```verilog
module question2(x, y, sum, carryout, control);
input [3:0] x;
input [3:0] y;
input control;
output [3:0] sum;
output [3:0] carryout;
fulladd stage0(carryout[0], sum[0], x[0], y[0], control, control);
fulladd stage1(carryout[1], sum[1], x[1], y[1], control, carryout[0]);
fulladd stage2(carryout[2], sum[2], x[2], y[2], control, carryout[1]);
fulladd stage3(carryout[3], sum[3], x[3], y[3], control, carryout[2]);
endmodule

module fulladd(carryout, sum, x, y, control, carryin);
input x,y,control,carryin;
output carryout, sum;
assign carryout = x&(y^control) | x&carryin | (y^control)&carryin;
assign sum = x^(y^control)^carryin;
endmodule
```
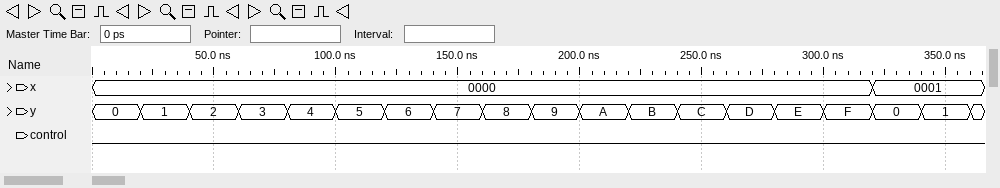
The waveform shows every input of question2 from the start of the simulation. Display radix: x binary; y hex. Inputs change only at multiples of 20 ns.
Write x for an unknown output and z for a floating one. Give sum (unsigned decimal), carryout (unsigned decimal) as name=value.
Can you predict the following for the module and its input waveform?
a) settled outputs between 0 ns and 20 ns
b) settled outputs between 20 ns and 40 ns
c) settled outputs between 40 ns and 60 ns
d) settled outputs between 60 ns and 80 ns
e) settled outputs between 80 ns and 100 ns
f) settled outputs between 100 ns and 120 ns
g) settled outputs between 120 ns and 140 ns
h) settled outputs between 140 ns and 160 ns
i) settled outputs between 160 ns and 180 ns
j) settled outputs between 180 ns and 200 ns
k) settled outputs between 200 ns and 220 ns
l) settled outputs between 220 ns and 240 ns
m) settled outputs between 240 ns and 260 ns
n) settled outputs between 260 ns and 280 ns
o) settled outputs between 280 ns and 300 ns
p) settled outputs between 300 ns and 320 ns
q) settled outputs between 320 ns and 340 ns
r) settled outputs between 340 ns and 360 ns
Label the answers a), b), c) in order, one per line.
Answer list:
a) sum=0, carryout=0
b) sum=1, carryout=0
c) sum=2, carryout=0
d) sum=3, carryout=0
e) sum=4, carryout=0
f) sum=5, carryout=0
g) sum=6, carryout=0
h) sum=7, carryout=0
i) sum=8, carryout=0
j) sum=9, carryout=0
k) sum=10, carryout=0
l) sum=11, carryout=0
m) sum=12, carryout=0
n) sum=13, carryout=0
o) sum=14, carryout=0
p) sum=15, carryout=0
q) sum=1, carryout=0
r) sum=2, carryout=1
